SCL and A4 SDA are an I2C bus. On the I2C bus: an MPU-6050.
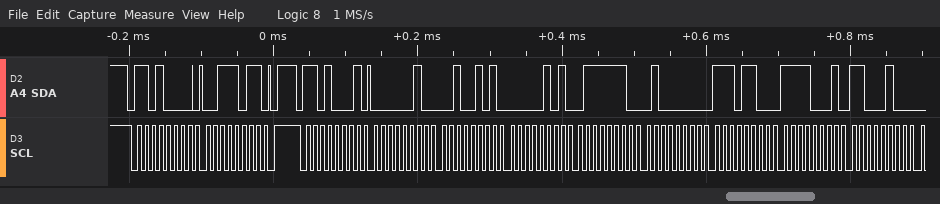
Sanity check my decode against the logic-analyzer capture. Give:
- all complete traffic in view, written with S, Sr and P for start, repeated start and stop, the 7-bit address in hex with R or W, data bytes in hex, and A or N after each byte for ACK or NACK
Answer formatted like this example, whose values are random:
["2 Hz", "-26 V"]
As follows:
["S 68W A 3B A P S 68R A 02 A 25 A 05 A 7E A 40 A EC A F1 A C4 A"]
